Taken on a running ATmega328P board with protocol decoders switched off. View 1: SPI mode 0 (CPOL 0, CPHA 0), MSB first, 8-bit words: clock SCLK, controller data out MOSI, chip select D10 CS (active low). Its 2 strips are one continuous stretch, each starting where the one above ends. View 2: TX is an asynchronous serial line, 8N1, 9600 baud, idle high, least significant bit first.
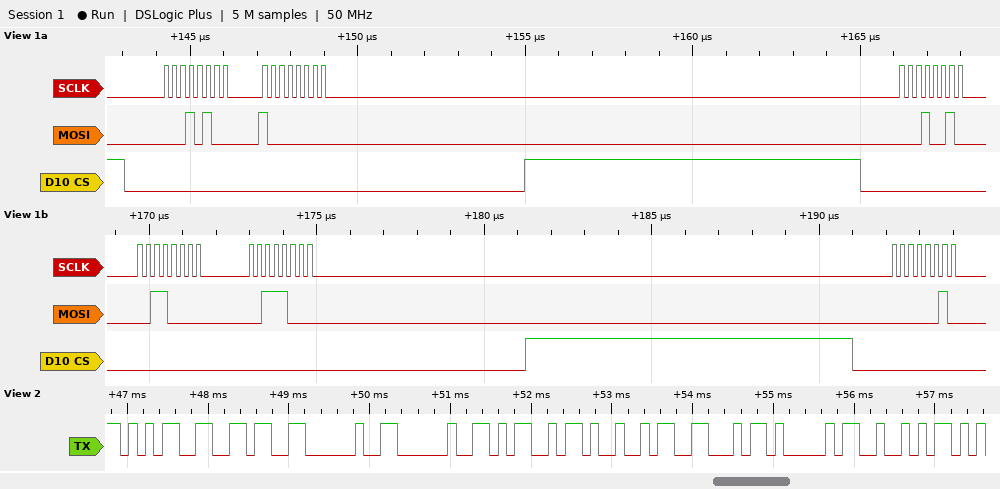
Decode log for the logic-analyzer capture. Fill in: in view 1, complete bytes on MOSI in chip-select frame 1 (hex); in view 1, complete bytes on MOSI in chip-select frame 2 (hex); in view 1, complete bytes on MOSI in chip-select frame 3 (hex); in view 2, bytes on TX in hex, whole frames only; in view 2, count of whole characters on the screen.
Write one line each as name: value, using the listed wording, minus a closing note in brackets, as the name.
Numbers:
in view 1, complete bytes on MOSI in chip-select frame 1: 14 80
in view 1, complete bytes on MOSI in chip-select frame 2: 12 30 38
in view 1, complete bytes on MOSI in chip-select frame 3: 02
in view 2, bytes on TX in hex, whole frames only: 35 36 20 20 4D 49 46 41 52
in view 2, count of whole characters on the screen: 9
